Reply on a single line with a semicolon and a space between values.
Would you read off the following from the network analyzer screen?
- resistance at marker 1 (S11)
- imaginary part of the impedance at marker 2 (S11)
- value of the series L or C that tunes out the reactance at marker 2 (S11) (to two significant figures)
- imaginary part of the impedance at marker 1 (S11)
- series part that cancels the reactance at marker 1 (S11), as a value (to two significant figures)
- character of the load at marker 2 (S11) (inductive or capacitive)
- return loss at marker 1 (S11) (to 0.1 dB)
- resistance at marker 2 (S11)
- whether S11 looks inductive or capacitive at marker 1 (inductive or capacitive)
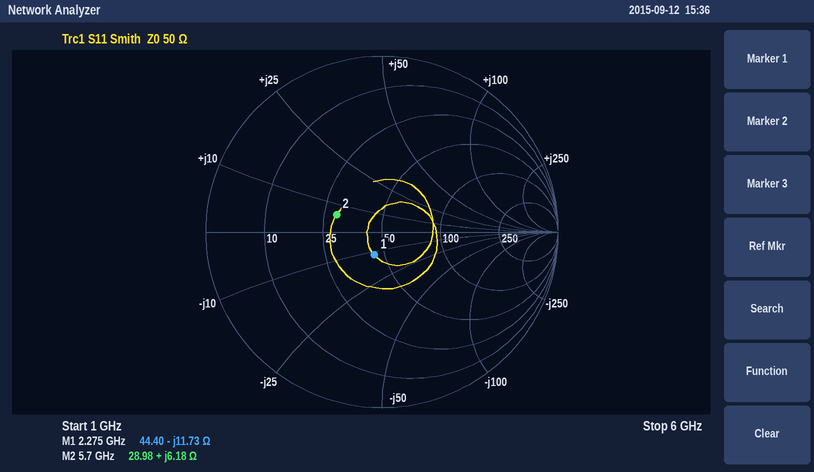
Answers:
44.40 Ω; +6.18 Ω; 4.5 pF; -11.73 Ω; 820 pH; inductive; 17.3 dB; 28.98 Ω; capacitive
